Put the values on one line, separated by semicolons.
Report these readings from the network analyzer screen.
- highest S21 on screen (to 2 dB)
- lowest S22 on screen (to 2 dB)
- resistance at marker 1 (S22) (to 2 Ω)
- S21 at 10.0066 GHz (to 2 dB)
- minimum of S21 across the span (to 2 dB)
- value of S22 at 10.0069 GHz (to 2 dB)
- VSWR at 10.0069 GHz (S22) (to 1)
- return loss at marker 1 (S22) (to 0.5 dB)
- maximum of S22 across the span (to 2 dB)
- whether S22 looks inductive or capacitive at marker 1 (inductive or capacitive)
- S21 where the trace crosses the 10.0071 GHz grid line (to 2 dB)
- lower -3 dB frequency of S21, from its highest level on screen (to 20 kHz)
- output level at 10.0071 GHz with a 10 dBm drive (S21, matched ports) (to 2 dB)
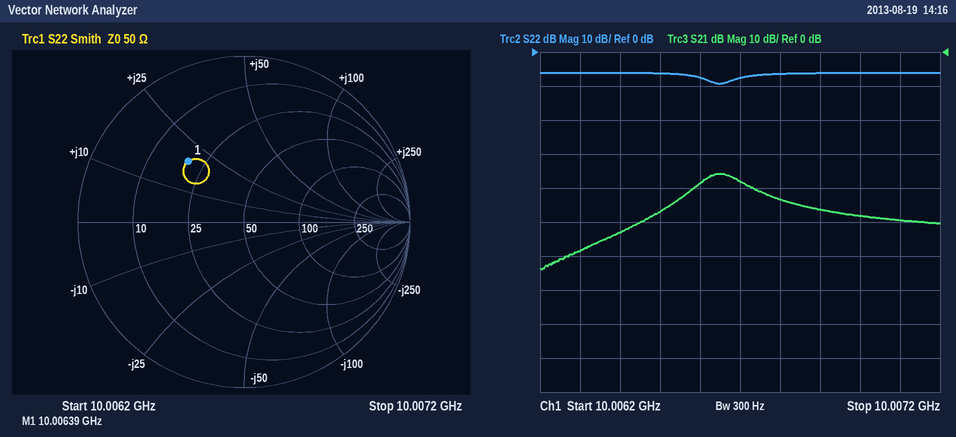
-36 dB; -10 dB; 20 Ω; -38 dB; -64 dB; -6 dB; 3; 6.0 dB; -6 dB; inductive; -50 dB; 10.00660 GHz; -40 dBm
